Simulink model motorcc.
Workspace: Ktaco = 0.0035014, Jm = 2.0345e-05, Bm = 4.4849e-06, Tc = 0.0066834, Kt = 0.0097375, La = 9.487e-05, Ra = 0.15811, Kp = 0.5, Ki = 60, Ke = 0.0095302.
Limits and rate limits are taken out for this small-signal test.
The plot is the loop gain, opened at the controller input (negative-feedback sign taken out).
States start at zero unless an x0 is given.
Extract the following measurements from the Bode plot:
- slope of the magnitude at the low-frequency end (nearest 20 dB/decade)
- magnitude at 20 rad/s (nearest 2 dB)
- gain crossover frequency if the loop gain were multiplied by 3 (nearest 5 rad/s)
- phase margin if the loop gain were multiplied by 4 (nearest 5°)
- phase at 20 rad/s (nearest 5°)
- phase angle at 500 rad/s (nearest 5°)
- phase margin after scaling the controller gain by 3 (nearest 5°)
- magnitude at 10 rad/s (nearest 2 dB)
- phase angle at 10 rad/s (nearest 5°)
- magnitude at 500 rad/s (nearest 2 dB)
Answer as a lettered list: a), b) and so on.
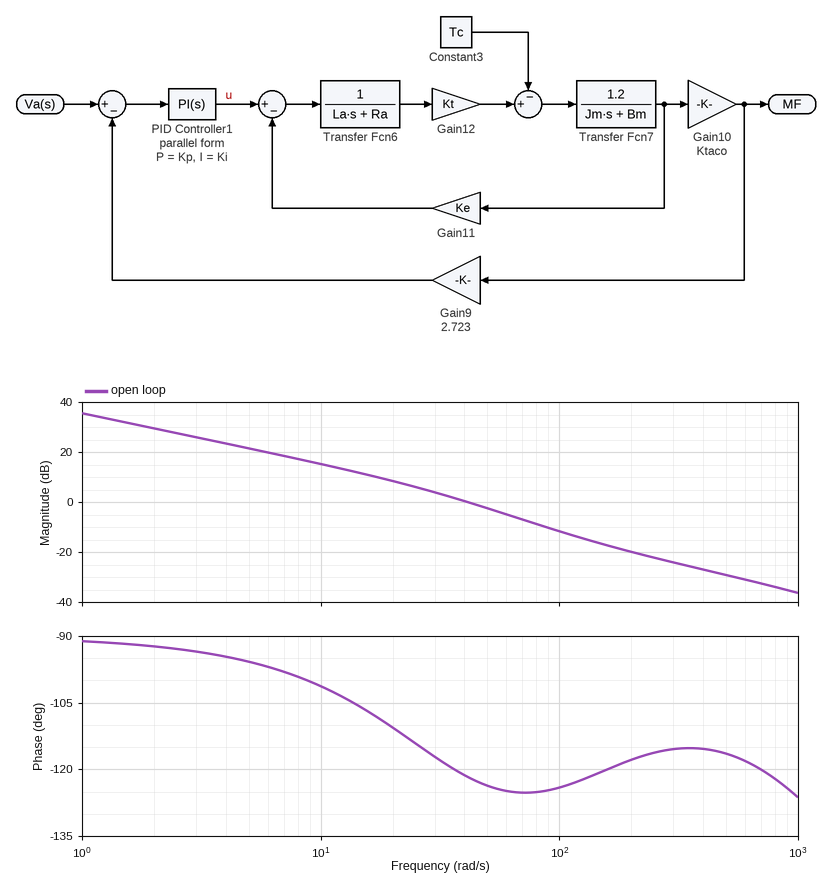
a) -20 dB/decade
b) 8 dB
c) 85 rad/s
d) 55°
e) -110°
f) -115°
g) 55°
h) 16 dB
i) -100°
j) -30 dB
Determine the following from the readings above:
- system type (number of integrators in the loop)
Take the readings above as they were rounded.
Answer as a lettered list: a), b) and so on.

a) 1
